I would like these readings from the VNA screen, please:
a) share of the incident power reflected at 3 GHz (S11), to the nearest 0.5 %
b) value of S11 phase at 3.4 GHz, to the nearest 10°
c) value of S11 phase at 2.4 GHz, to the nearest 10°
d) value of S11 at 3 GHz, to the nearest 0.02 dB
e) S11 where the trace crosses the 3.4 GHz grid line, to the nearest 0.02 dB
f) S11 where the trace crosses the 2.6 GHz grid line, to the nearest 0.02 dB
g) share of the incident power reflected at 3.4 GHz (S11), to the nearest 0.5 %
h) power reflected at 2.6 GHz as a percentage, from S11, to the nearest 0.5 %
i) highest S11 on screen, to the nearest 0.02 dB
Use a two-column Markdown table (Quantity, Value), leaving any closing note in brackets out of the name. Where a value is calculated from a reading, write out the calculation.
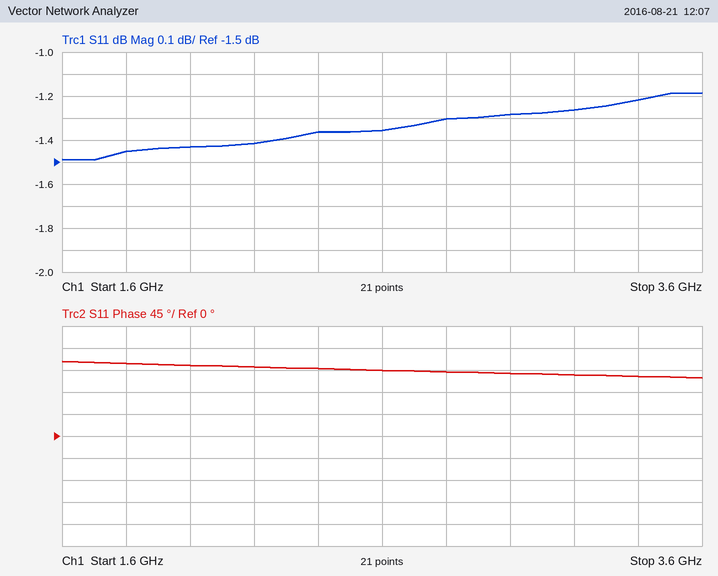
| Quantity | Value |
|---|---|
| share of the incident power reflected at 3 GHz (S11), to the nearest 0.5 % | 10^(-1.28/10) ≈ 74.5 % |
| value of S11 phase at 3.4 GHz, to the nearest 10° | 120° |
| value of S11 phase at 2.4 GHz, to the nearest 10° | 140° |
| value of S11 at 3 GHz, to the nearest 0.02 dB | -1.28 dB |
| S11 where the trace crosses the 3.4 GHz grid line, to the nearest 0.02 dB | -1.22 dB |
| S11 where the trace crosses the 2.6 GHz grid line, to the nearest 0.02 dB | -1.36 dB |
| share of the incident power reflected at 3.4 GHz (S11), to the nearest 0.5 % | 10^(-1.22/10) ≈ 75.5 % |
| power reflected at 2.6 GHz as a percentage, from S11, to the nearest 0.5 % | 10^(-1.36/10) ≈ 73.1 %, so 73.0 % to the nearest 0.5 % |
| highest S11 on screen, to the nearest 0.02 dB | -1.18 dB |
